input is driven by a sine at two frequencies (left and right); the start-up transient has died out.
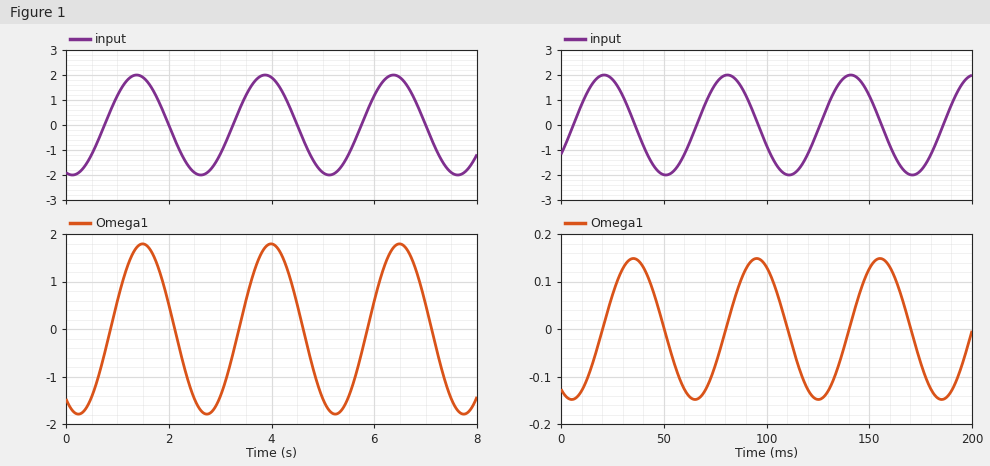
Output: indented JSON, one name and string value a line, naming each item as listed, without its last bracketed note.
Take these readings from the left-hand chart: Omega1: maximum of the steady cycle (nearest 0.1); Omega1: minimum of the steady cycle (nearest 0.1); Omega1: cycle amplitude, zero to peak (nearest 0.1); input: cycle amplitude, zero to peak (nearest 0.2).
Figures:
{
  "Omega1: maximum of the steady cycle": "1.8",
  "Omega1: minimum of the steady cycle": "-1.8",
  "Omega1: cycle amplitude, zero to peak": "1.8",
  "input: cycle amplitude, zero to peak": "2.0"
}
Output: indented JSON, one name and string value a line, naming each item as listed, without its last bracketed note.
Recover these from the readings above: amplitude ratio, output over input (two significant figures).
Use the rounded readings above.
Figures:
{
  "amplitude ratio, output over input": "0.90"
}
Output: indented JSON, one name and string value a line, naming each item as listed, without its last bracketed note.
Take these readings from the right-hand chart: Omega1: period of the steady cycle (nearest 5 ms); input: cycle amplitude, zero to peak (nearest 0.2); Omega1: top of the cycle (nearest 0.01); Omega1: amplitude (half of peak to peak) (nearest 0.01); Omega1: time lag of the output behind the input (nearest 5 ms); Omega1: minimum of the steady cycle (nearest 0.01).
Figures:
{
  "Omega1: period of the steady cycle": "60 ms",
  "input: cycle amplitude, zero to peak": "2.0",
  "Omega1: top of the cycle": "0.15",
  "Omega1: amplitude (half of peak to peak)": "0.15",
  "Omega1: time lag of the output behind the input": "15 ms",
  "Omega1: minimum of the steady cycle": "-0.15"
}
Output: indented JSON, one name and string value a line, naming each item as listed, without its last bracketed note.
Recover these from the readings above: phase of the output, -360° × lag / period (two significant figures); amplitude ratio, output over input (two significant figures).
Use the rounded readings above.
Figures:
{
  "phase of the output, -360° × lag / period": "-90°",
  "amplitude ratio, output over input": "0.075"
}
